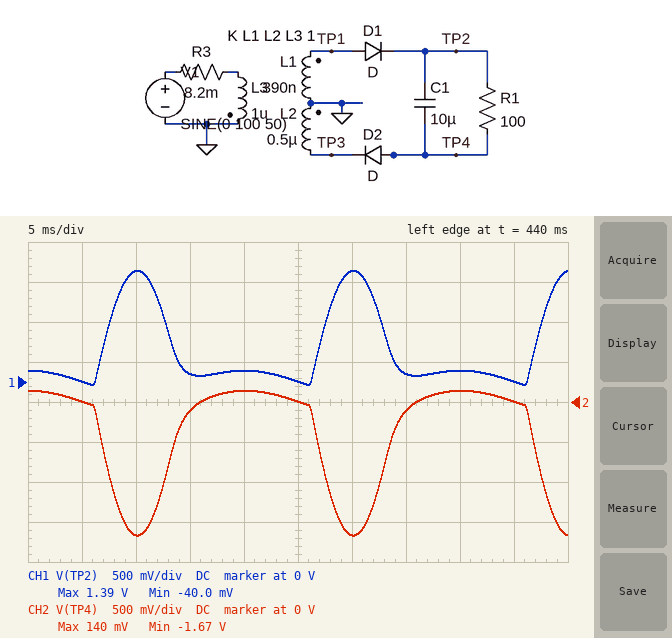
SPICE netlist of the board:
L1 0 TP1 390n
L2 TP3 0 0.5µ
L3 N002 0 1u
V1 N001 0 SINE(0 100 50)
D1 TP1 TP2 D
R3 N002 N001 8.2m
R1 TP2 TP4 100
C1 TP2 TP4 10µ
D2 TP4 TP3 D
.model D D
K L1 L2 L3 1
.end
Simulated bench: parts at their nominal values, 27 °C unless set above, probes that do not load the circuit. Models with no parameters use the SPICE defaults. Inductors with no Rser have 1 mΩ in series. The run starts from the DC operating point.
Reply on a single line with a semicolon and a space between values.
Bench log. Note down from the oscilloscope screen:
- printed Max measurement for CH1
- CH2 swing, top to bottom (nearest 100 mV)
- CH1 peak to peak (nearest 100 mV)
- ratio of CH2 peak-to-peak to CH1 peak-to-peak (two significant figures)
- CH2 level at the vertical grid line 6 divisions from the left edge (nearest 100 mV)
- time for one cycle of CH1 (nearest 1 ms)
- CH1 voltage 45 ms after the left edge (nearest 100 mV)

1.39 V; 1.8 V; 1.4 V; 1.3; -1.7 V; 20 ms; 0 V
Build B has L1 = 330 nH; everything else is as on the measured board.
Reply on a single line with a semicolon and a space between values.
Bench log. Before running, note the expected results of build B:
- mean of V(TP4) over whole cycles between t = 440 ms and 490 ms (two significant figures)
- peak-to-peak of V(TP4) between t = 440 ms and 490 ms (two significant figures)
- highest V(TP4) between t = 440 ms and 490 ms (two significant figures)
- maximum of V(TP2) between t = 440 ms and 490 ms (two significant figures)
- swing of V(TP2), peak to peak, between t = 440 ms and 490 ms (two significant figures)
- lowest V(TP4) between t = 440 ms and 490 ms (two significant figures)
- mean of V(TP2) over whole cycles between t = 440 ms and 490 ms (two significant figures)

-390 mV; 1.9 V; 230 mV; 1.2 V; 1.3 V; -1.7 V; 390 mV
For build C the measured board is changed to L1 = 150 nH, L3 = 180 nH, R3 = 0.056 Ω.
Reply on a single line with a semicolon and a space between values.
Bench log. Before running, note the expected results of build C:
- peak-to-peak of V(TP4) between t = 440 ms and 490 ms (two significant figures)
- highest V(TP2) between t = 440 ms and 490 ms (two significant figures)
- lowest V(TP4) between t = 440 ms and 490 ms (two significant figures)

75 mV; 37 mV; -37 mV
